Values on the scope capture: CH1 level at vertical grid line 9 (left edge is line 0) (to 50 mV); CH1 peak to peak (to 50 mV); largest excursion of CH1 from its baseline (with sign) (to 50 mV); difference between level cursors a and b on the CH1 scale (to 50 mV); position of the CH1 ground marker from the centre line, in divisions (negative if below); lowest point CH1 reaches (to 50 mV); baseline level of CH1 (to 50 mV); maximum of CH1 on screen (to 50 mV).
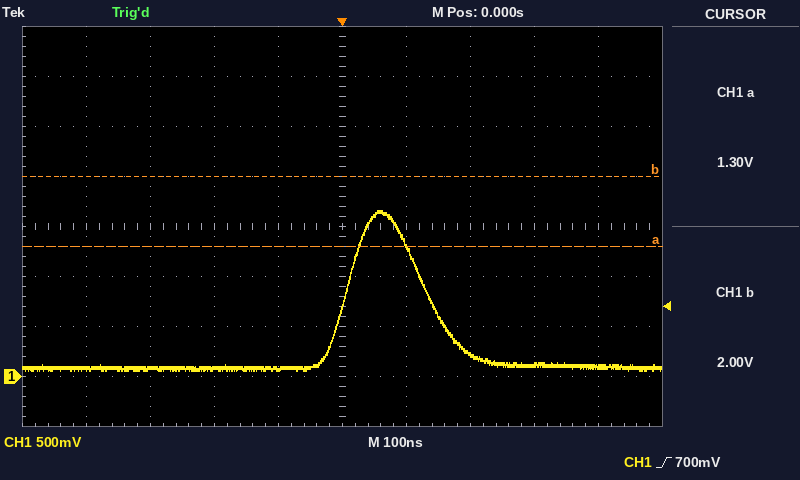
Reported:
100 mV
1.60 V
+1.55 V
700 mV
-3.0 div
50 mV
100 mV
1.65 V
